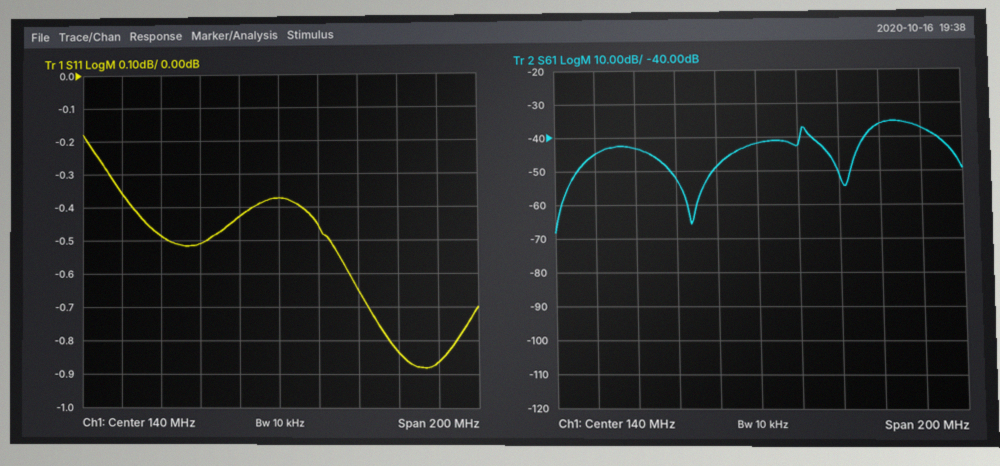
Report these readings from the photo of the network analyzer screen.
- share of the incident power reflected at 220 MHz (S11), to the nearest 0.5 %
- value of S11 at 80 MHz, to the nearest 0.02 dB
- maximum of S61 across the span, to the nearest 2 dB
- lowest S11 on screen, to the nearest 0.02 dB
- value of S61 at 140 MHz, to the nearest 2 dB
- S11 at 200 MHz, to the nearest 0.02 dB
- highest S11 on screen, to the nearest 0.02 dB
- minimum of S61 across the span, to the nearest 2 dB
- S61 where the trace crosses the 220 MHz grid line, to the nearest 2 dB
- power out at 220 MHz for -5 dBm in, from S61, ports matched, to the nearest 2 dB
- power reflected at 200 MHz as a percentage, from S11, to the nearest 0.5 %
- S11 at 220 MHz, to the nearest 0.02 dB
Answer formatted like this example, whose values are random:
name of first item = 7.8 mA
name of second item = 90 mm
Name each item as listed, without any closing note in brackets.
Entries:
share of the incident power reflected at 220 MHz (S11), to the nearest 0.5 % = 82.0 %
value of S11 at 80 MHz, to the nearest 0.02 dB = -0.48 dB
maximum of S61 across the span, to the nearest 2 dB = -36 dB
lowest S11 on screen, to the nearest 0.02 dB = -0.88 dB
value of S61 at 140 MHz, to the nearest 2 dB = -42 dB
S11 at 200 MHz, to the nearest 0.02 dB = -0.84 dB
highest S11 on screen, to the nearest 0.02 dB = -0.18 dB
minimum of S61 across the span, to the nearest 2 dB = -68 dB
S61 where the trace crosses the 220 MHz grid line, to the nearest 2 dB = -38 dB
power out at 220 MHz for -5 dBm in, from S61, ports matched, to the nearest 2 dB = -42 dBm
power reflected at 200 MHz as a percentage, from S11, to the nearest 0.5 % = 82.5 %
S11 at 220 MHz, to the nearest 0.02 dB = -0.86 dB
